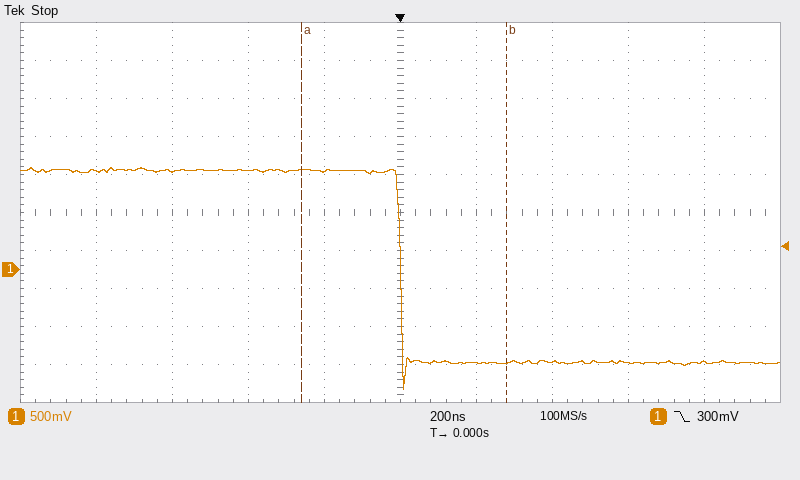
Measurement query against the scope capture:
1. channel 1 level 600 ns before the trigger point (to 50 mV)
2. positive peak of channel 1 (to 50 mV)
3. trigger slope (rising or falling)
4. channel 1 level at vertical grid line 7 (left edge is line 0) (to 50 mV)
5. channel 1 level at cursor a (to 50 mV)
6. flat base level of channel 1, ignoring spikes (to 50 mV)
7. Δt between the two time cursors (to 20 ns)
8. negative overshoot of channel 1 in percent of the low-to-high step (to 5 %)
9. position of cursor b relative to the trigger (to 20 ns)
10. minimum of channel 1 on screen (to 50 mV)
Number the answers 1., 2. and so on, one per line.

1. 1.30 V
2. 1.35 V
3. falling
4. -1.20 V
5. 1.30 V
6. -1.20 V
7. 540 ns
8. 15 %
9. +280 ns
10. -1.60 V
